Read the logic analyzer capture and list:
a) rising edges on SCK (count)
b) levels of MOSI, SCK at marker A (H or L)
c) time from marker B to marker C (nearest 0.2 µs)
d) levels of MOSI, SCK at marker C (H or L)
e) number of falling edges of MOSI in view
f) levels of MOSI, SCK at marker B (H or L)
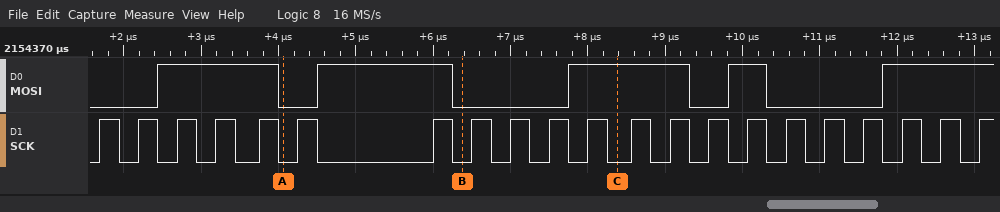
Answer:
21
MOSI=L, SCK=L
2 µs
MOSI=H, SCK=L
4
MOSI=L, SCK=L
